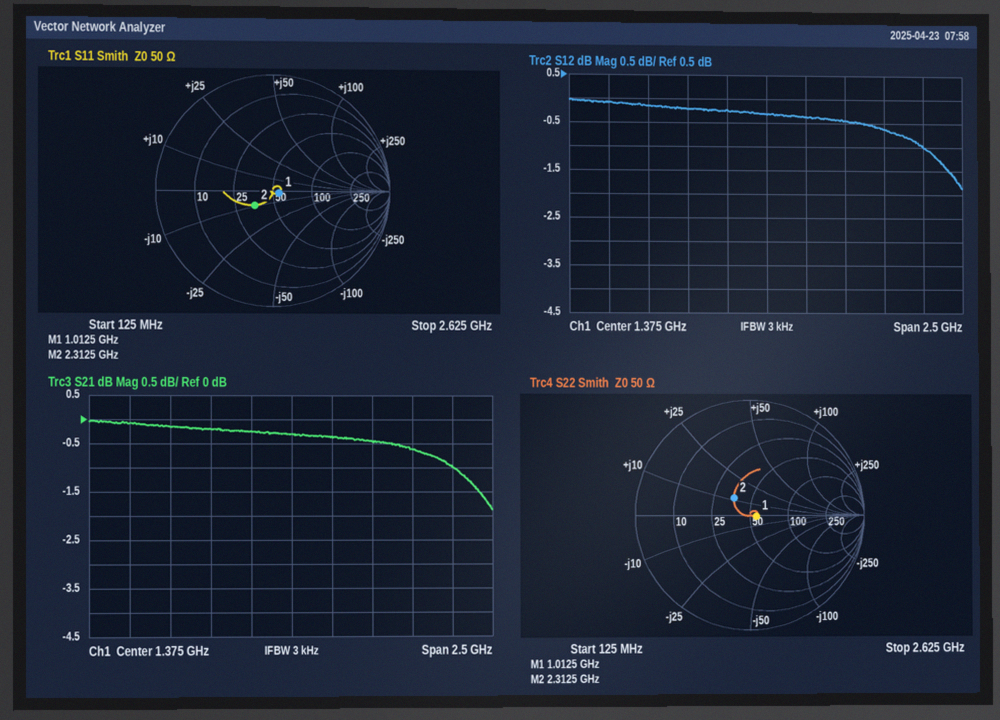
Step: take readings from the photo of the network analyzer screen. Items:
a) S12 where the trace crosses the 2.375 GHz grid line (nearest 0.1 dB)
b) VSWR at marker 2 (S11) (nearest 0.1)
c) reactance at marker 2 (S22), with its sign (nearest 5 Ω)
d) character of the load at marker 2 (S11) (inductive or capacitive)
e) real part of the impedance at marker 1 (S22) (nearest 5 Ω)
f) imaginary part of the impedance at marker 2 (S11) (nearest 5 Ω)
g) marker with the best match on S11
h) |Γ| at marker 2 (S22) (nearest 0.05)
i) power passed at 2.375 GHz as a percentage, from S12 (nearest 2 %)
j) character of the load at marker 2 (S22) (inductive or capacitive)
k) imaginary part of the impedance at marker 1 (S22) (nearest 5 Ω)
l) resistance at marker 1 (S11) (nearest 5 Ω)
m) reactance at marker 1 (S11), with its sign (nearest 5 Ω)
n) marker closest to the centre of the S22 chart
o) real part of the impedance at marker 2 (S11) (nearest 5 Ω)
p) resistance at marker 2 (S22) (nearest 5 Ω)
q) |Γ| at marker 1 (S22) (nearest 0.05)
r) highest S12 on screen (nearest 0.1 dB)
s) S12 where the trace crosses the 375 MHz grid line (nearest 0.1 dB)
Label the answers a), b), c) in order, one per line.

a) -1.0 dB
b) 1.5
c) +10 Ω
d) capacitive
e) 55 Ω
f) -10 Ω
g) marker 1
h) 0.20
i) 80 %
j) inductive
k) 0 Ω
l) 55 Ω
m) 0 Ω
n) marker 1
o) 35 Ω
p) 35 Ω
q) 0.05
r) 0.0 dB
s) -0.1 dB
